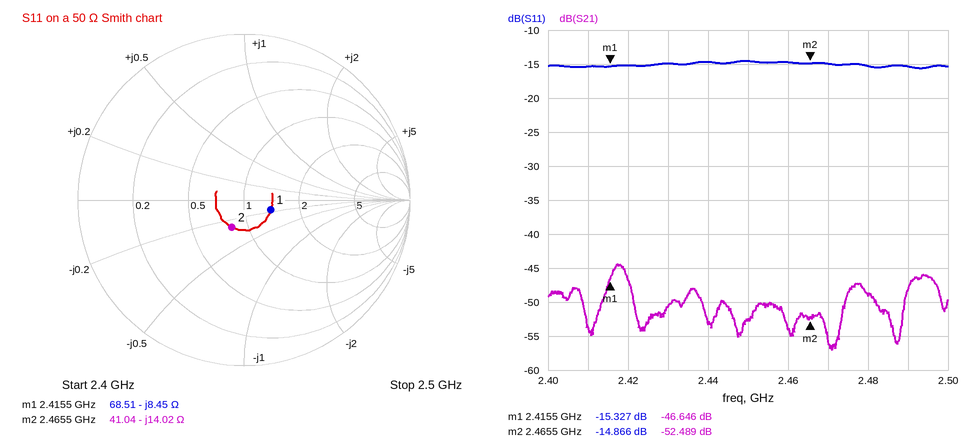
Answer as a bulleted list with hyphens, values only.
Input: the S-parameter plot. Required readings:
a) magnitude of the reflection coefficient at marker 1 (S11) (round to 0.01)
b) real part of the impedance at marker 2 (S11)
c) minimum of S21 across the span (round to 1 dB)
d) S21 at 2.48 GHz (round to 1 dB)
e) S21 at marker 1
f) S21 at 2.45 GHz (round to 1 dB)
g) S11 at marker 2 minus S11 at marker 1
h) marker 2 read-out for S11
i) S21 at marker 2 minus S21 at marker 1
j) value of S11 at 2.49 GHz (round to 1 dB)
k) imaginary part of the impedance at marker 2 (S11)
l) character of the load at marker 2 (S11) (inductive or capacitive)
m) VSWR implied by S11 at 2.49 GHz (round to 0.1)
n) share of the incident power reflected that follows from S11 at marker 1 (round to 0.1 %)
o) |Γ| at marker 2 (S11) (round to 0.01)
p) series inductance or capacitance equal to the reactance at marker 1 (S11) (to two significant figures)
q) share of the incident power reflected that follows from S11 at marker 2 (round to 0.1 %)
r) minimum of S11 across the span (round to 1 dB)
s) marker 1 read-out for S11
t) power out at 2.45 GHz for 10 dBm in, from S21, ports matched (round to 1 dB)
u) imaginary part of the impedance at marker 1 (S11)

- 0.17
- 41.04 Ω
- -57 dB
- -49 dB
- -46.646 dB
- -53 dB
- 0.461 dB
- -14.866 dB
- -5.843 dB
- -15 dB
- -14.02 Ω
- capacitive
- 1.4
- 2.9 %
- 0.18
- 7.8 pF
- 3.3 %
- -16 dB
- -15.327 dB
- -43 dBm
- -8.45 Ω
